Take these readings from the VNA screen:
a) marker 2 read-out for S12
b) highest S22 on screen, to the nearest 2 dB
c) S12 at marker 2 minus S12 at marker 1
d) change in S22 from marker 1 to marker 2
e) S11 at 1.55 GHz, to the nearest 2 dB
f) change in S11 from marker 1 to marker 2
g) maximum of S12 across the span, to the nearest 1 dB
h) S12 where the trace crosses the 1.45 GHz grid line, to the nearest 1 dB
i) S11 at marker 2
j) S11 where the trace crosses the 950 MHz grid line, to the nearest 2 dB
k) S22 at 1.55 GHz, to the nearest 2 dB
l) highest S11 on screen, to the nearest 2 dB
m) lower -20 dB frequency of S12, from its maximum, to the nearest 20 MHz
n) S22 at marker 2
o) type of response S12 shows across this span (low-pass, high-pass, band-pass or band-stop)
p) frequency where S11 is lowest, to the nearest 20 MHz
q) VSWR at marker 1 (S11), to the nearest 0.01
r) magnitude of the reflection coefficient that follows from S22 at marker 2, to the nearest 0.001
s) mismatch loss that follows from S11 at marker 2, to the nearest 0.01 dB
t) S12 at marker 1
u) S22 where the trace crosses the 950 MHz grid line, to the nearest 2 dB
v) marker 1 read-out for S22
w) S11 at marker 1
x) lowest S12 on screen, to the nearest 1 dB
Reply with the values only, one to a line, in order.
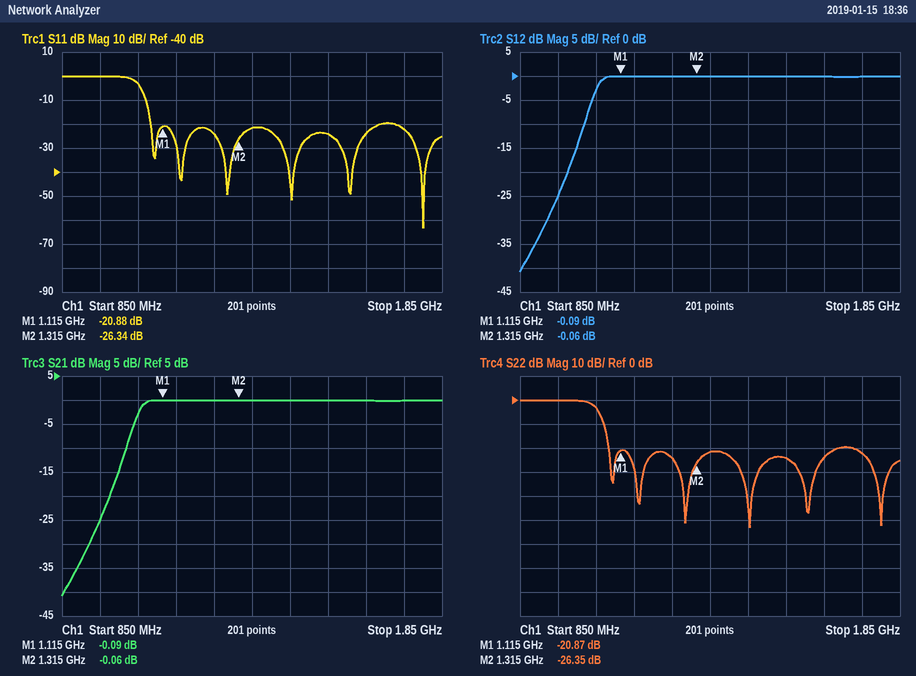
-0.06 dB
0 dB
0.03 dB
-5.48 dB
-24 dB
-5.46 dB
0 dB
0 dB
-26.34 dB
0 dB
-24 dB
0 dB
980 MHz
-26.35 dB
high-pass
1.80 GHz
1.20
0.048
0.01 dB
-0.09 dB
0 dB
-20.87 dB
-20.88 dB
-41 dB
